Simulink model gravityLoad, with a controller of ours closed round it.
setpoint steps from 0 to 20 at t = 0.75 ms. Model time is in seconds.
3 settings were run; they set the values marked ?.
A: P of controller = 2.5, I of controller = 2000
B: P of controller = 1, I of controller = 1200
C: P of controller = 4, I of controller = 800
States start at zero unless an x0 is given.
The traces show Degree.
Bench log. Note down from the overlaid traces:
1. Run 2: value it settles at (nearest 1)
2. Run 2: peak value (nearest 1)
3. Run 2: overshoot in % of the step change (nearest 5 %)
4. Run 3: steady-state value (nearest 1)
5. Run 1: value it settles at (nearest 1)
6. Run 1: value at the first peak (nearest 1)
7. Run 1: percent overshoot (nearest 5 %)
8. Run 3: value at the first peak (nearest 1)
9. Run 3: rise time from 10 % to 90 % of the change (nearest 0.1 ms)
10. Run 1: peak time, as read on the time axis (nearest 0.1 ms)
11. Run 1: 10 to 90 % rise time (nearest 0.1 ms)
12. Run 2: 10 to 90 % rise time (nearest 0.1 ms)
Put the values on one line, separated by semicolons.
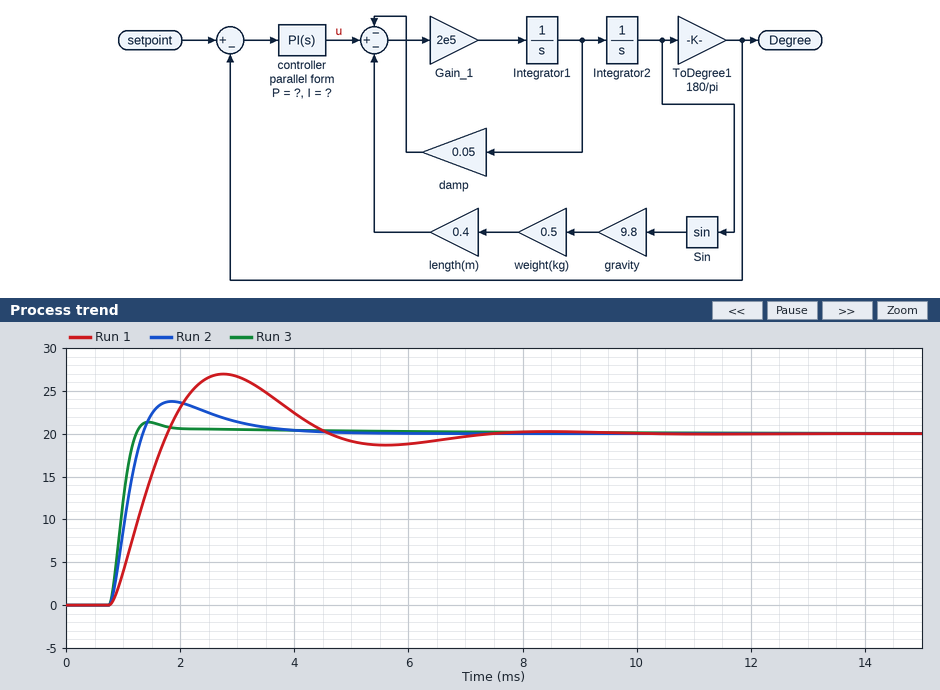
20; 24; 20 %; 20; 20; 27; 35 %; 21; 0.3 ms; 2.8 ms; 0.7 ms; 0.4 ms
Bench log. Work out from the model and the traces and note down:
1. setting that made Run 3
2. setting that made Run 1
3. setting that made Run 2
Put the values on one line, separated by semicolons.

C; B; A
